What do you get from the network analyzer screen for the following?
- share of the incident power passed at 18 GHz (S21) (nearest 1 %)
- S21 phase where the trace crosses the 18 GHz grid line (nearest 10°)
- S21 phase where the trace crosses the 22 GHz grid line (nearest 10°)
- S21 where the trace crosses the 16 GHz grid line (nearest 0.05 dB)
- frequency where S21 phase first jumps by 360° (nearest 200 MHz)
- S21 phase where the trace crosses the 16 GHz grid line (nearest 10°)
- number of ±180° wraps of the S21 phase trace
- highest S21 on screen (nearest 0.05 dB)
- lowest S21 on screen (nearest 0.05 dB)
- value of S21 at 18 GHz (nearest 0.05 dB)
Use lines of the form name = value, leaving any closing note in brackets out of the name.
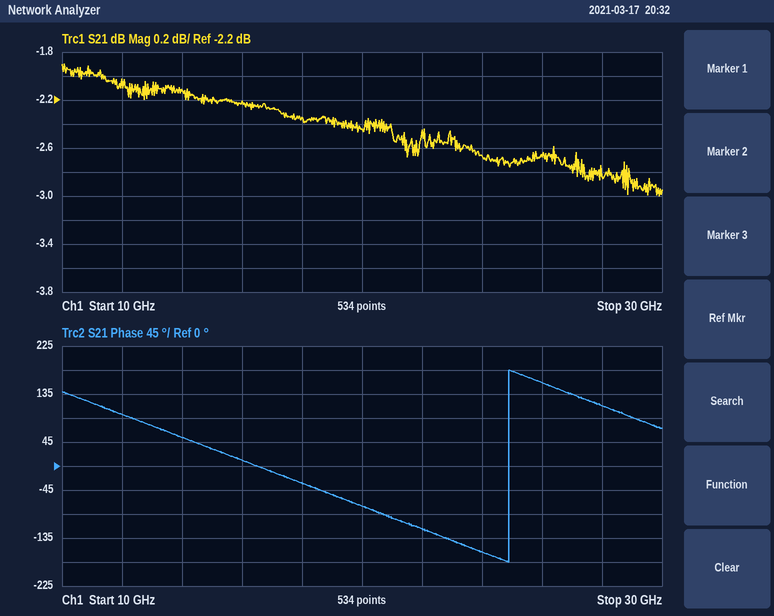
share of the incident power passed at 18 GHz (S21) = 58 %
S21 phase where the trace crosses the 18 GHz grid line = -30°
S21 phase where the trace crosses the 22 GHz grid line = -120°
S21 where the trace crosses the 16 GHz grid line = -2.20 dB
frequency where S21 phase first jumps by 360° = 24.8 GHz
S21 phase where the trace crosses the 16 GHz grid line = 10°
number of ±180° wraps of the S21 phase trace = 1
highest S21 on screen = -1.90 dB
lowest S21 on screen = -3.00 dB
value of S21 at 18 GHz = -2.35 dB
